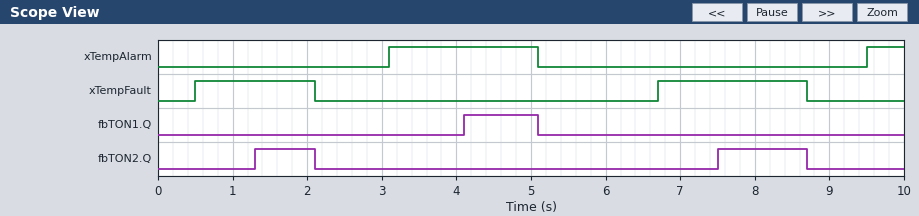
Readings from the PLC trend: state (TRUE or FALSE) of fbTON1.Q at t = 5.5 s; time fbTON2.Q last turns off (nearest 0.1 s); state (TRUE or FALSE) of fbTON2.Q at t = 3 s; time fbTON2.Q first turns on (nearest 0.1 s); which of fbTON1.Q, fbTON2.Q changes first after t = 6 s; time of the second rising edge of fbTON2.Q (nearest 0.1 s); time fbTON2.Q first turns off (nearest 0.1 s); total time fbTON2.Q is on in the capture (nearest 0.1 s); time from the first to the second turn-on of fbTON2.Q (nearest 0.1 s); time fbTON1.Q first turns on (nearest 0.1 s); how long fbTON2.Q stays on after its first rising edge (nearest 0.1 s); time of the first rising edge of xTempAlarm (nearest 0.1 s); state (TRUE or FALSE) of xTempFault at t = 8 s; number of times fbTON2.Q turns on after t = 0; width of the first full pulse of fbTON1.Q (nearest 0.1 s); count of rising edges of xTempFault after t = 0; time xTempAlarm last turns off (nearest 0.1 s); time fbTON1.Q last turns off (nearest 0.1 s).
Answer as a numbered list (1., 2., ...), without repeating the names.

1. FALSE
2. 8.7 s
3. FALSE
4. 1.3 s
5. fbTON2.Q
6. 7.5 s
7. 2.1 s
8. 2.0 s
9. 6.2 s
10. 4.1 s
11. 0.8 s
12. 3.1 s
13. TRUE
14. 2
15. 1.0 s
16. 2
17. 5.1 s
18. 5.1 s
